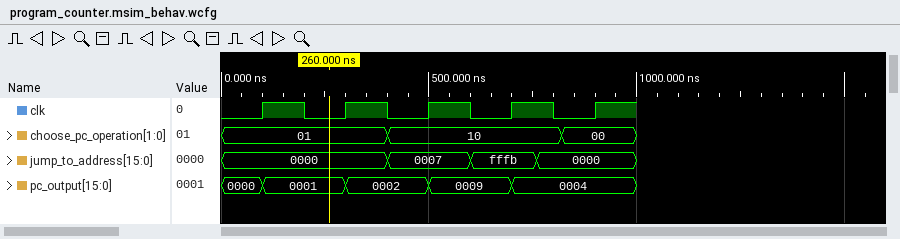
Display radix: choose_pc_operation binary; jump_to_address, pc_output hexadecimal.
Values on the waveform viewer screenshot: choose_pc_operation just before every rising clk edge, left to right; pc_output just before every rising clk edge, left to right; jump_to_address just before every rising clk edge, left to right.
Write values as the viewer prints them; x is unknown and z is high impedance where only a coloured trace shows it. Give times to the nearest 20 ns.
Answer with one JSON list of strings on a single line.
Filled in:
["01, 01, 10, 10, 00", "0000, 0001, 0002, 0009, 0004", "0000, 0000, 0007, fffb, 0000"]
